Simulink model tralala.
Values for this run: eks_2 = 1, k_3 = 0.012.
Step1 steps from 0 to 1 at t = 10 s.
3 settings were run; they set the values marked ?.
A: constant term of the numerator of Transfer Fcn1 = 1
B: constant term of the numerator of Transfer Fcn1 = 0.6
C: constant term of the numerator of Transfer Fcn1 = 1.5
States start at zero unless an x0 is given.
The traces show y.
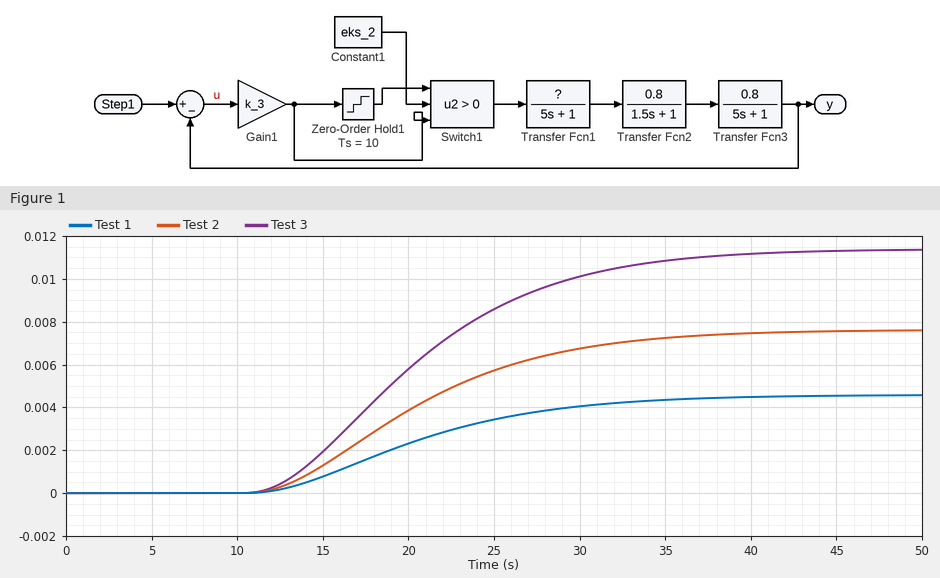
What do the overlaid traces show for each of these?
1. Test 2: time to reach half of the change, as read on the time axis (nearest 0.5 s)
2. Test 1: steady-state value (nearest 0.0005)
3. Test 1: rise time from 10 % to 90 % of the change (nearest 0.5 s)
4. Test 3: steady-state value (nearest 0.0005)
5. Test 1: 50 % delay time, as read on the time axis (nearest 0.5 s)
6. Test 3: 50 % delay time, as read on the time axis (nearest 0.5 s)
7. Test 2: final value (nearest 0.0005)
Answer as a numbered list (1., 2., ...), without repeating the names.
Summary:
1. 20.0 s
2. 0.0045
3. 17.0 s
4. 0.0115
5. 20.0 s
6. 20.0 s
7. 0.0075
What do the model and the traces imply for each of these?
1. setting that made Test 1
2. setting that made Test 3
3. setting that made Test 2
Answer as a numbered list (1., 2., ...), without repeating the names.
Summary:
1. B
2. C
3. A
